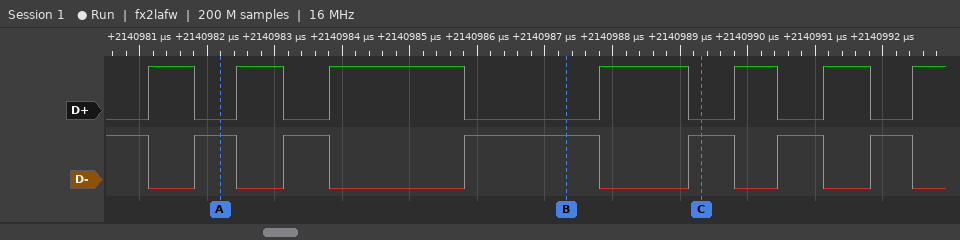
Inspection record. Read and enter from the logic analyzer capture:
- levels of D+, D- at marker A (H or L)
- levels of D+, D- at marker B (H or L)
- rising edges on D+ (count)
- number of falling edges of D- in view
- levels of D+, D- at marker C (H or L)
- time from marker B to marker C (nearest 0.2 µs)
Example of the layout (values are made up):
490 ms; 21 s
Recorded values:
D+=L, D-=H; D+=L, D-=H; 7; 7; D+=L, D-=H; 2 µs
